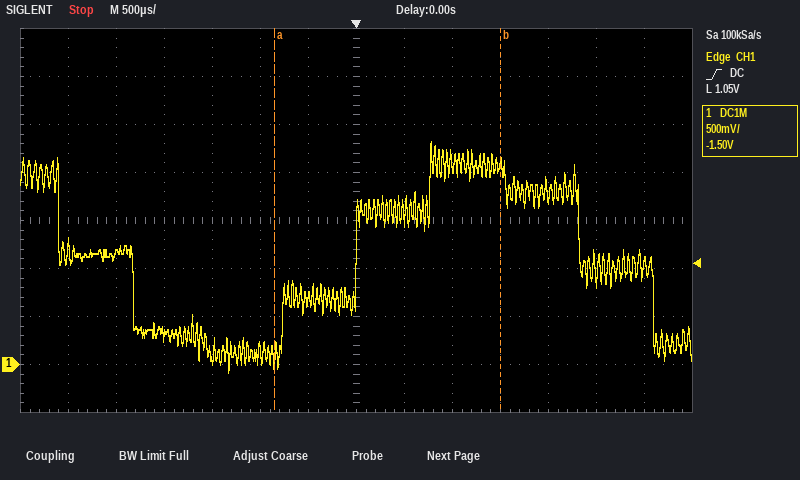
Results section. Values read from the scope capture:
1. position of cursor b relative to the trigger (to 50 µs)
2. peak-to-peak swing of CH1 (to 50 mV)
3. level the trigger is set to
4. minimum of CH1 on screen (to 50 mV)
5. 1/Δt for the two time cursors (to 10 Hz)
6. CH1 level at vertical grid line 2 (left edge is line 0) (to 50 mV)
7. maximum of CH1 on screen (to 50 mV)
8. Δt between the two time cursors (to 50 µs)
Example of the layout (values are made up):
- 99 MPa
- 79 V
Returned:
- +1.50 ms
- 2.40 V
- 1.05 V
- -100 mV
- 430 Hz
- 1.15 V
- 2.30 V
- 2.35 ms
